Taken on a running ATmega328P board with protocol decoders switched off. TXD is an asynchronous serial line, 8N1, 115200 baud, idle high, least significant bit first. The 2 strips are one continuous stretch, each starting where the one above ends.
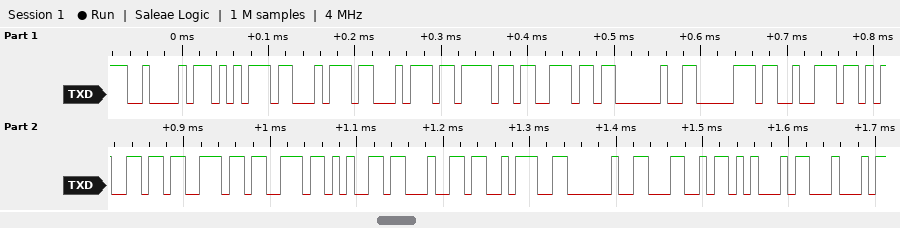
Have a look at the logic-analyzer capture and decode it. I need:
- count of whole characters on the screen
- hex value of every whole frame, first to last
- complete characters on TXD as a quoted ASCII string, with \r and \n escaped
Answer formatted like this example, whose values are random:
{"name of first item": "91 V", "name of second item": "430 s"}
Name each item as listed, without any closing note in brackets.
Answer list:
{"count of whole characters on the screen": "19", "hex value of every whole frame, first to last": "0x42 0x75 0x74 0x74 0x6F 0x6E 0x20 0x70 0x72 0x65 0x73 0x73 0x65 0x64 0x3A 0x20 0x4C 0x45 0x44", "complete characters on TXD as a quoted ASCII string, with \\r and \\n escaped": "\"Button pressed: LED\""}
